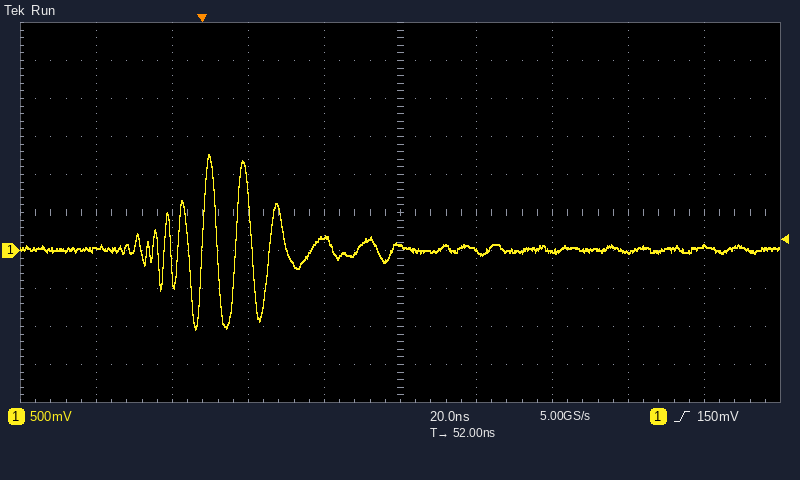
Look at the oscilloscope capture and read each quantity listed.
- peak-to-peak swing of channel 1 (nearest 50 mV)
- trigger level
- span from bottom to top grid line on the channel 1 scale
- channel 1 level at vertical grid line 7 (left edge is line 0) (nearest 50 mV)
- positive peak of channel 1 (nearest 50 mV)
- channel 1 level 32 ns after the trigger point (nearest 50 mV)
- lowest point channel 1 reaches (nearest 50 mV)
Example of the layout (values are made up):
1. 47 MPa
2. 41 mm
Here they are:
1. 2.30 V
2. 150 mV
3. 5 V
4. 0 mV
5. 1.25 V
6. 200 mV
7. -1.05 V
